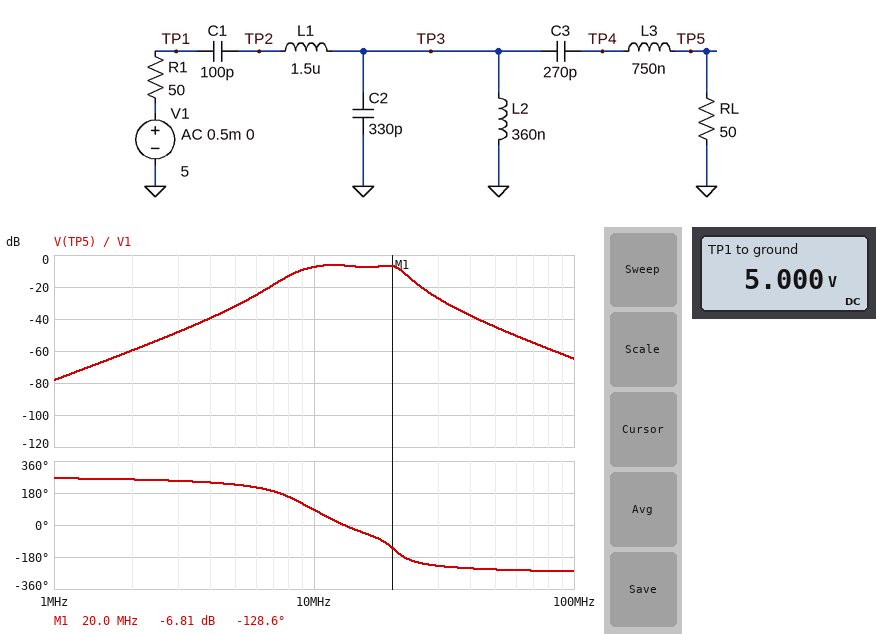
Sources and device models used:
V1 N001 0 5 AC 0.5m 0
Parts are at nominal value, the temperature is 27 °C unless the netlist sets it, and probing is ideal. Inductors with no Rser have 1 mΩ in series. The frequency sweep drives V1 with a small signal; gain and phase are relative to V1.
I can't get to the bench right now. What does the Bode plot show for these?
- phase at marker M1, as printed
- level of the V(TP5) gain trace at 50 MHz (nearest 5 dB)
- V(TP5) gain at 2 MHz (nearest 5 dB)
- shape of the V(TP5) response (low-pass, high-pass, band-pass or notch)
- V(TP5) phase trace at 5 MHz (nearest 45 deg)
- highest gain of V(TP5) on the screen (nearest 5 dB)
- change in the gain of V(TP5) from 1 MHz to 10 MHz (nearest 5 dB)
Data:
-128.6 deg
-45 dB
-60 dB
band-pass
225 deg
-5 dB
70 dB
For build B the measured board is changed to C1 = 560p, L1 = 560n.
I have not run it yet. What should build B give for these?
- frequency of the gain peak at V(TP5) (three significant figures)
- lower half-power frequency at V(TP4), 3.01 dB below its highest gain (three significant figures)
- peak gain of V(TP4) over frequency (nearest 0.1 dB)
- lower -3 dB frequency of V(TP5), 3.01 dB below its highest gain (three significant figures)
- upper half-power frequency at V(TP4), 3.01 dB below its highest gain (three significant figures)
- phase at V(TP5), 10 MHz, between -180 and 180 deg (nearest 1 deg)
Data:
20.0 MHz
15.4 MHz
0.7 dB
7.53 MHz
24.2 MHz
35 deg
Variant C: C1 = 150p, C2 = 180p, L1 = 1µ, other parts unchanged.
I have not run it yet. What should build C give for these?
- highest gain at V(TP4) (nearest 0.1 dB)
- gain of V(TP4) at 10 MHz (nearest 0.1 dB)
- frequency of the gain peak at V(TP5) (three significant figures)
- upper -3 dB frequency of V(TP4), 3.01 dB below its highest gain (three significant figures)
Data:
2.6 dB
-4.9 dB
27.1 MHz
29.7 MHz
